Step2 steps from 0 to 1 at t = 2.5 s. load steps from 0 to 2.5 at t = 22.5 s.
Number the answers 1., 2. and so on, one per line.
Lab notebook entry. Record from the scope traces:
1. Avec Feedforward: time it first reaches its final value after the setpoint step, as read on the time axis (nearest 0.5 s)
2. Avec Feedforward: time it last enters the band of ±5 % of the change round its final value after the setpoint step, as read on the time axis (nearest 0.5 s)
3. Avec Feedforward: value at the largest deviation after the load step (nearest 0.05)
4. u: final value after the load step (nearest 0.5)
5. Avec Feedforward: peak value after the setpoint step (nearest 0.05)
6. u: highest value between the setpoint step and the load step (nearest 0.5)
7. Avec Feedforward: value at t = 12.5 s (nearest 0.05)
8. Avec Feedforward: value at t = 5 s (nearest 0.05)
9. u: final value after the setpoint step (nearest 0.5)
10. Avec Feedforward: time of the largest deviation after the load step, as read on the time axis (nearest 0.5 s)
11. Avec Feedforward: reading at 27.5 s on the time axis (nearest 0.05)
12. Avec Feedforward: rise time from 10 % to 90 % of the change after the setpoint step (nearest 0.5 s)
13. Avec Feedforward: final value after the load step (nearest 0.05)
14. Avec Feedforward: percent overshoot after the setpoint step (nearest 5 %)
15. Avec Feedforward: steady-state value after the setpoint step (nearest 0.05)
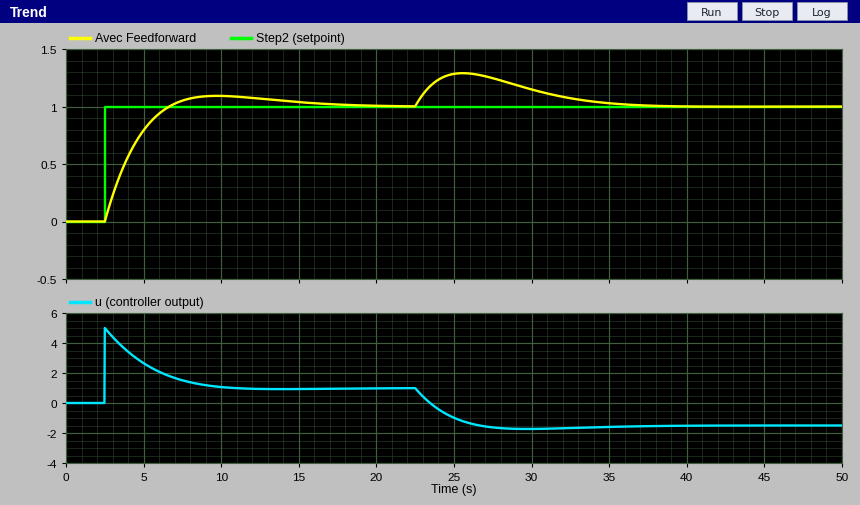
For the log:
1. 6.5 s
2. 14.0 s
3. 1.30
4. -1.5
5. 1.10
6. 5.0
7. 1.05
8. 0.80
9. 1.0
10. 25.5 s
11. 1.25
12. 3.0 s
13. 1.00
14. 10 %
15. 1.00
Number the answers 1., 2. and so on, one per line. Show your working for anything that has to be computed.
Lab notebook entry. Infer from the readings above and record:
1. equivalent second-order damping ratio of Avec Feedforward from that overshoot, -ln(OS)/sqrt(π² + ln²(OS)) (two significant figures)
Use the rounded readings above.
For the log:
1. ln(0.1) = -2.303; 2.303 / sqrt(9.870 + 5.302) = 0.59
